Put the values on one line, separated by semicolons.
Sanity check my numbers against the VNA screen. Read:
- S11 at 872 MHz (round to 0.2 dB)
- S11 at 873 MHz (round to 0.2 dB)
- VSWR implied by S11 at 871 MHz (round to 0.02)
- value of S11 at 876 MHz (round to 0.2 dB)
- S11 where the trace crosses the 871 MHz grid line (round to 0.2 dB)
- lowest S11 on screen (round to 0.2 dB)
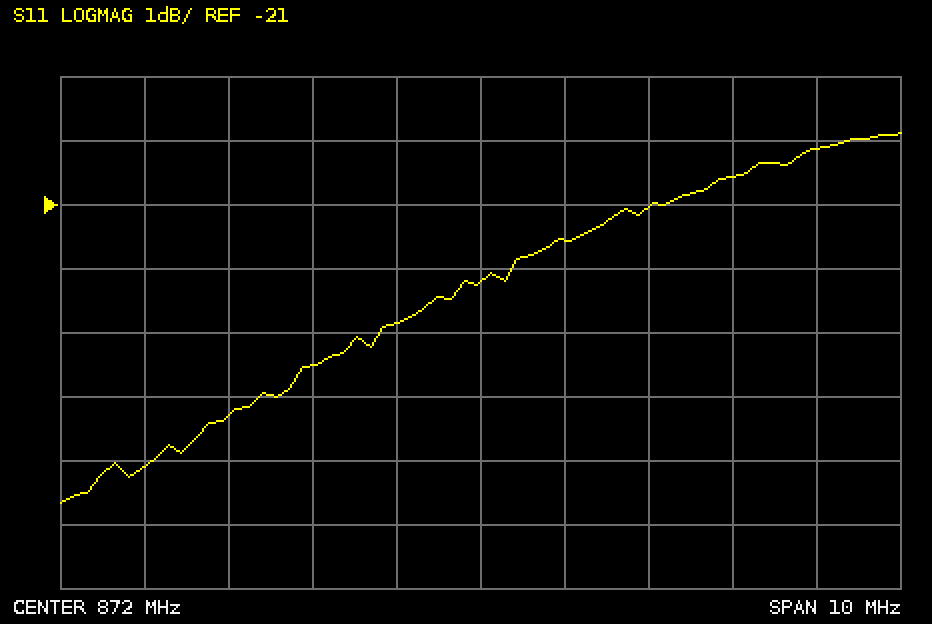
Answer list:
-22.2 dB; -21.6 dB; 1.16; -20.2 dB; -22.8 dB; -25.6 dB
